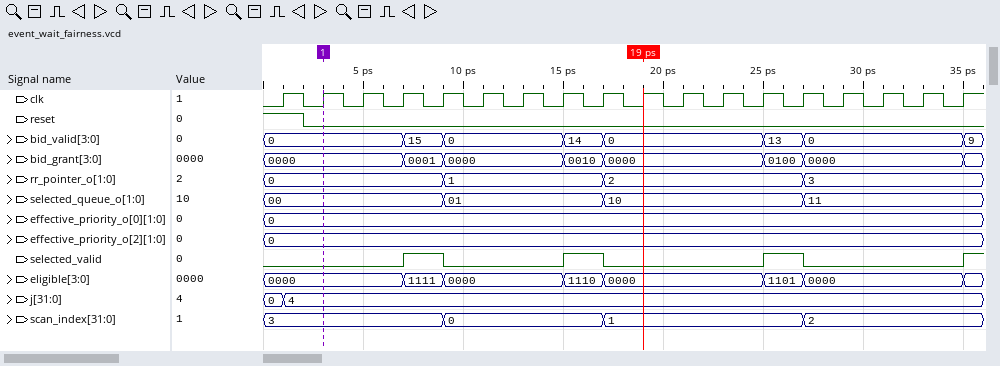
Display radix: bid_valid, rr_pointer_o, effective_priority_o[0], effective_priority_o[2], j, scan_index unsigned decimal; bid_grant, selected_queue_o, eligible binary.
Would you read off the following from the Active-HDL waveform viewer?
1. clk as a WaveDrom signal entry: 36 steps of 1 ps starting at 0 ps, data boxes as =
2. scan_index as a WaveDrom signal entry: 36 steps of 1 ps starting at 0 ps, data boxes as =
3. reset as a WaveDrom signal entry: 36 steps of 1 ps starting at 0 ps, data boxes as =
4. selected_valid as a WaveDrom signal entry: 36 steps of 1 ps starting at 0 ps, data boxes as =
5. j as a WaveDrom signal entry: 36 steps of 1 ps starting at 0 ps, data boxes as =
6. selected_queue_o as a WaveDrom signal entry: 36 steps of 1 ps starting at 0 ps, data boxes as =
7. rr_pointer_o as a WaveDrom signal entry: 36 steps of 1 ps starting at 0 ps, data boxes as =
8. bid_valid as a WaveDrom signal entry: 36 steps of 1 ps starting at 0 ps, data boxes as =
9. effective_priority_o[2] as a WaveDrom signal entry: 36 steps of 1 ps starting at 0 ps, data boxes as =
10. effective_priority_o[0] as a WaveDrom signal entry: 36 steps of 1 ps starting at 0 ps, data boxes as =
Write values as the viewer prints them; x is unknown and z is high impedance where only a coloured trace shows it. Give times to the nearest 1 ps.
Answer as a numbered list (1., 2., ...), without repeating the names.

1. {name: 'clk', wave: '010101010101010101010101010101010101'}
2. {name: 'scan_index', wave: '=........=.......=.........=........', data: '3 0 1 2'}
3. {name: 'reset', wave: '1.0.................................'}
4. {name: 'selected_valid', wave: '0......1.0.....1.0.......1.0.......1'}
5. {name: 'j', wave: '==..................................', data: '0 4'}
6. {name: 'selected_queue_o', wave: '=........=.......=.........=........', data: '00 01 10 11'}
7. {name: 'rr_pointer_o', wave: '=........=.......=.........=........', data: '0 1 2 3'}
8. {name: 'bid_valid', wave: '=......=.=.....=.=.......=.=.......=', data: '0 15 0 14 0 13 0 9'}
9. {name: 'effective_priority_o[2]', wave: '=...................................', data: '0'}
10. {name: 'effective_priority_o[0]', wave: '=...................................', data: '0'}
